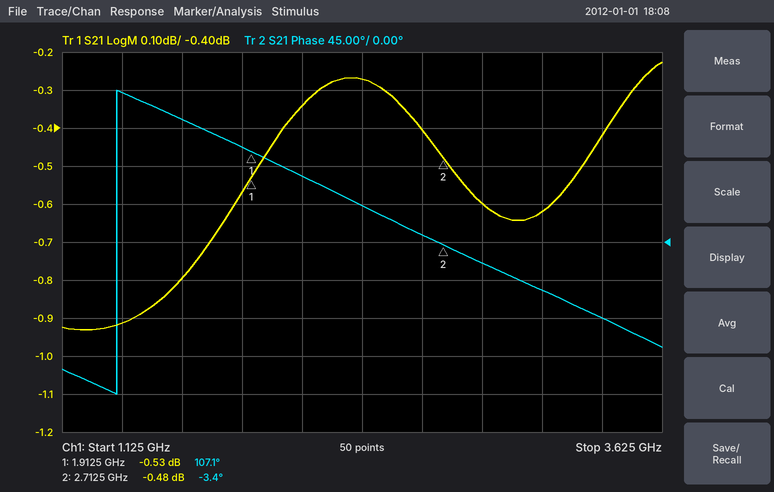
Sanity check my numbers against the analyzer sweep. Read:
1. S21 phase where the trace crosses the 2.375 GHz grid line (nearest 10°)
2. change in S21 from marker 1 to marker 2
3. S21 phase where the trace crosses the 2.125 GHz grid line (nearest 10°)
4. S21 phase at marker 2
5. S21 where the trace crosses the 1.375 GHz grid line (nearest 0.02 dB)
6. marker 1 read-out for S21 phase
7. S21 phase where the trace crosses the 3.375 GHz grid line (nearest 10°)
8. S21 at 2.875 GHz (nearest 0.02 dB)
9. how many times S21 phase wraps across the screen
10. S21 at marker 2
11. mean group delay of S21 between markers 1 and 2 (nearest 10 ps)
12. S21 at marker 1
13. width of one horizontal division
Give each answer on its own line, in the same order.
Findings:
40°
0.05 dB
80°
-3.4°
-0.92 dB
107.1°
-90°
-0.60 dB
1
-0.48 dB
380 ps
-0.53 dB
250 MHz
